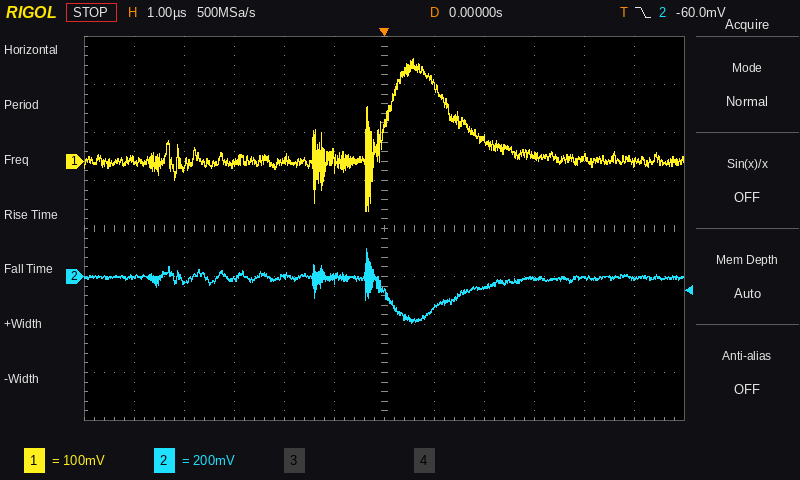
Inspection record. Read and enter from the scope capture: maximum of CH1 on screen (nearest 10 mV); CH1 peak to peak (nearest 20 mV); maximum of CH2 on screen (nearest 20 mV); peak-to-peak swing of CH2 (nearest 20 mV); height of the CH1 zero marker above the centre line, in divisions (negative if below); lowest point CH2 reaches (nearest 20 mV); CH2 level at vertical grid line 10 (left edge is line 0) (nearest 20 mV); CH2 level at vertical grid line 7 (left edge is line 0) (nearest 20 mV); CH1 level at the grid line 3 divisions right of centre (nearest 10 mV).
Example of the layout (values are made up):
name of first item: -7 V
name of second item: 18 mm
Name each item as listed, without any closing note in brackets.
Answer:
maximum of CH1 on screen: 210 mV
CH1 peak to peak: 320 mV
maximum of CH2 on screen: 120 mV
peak-to-peak swing of CH2: 320 mV
height of the CH1 zero marker above the centre line, in divisions: +1.4 div
lowest point CH2 reaches: -200 mV
CH2 level at vertical grid line 10 (left edge is line 0): 0 mV
CH2 level at vertical grid line 7 (left edge is line 0): -140 mV
CH1 level at the grid line 3 divisions right of centre: 10 mV
